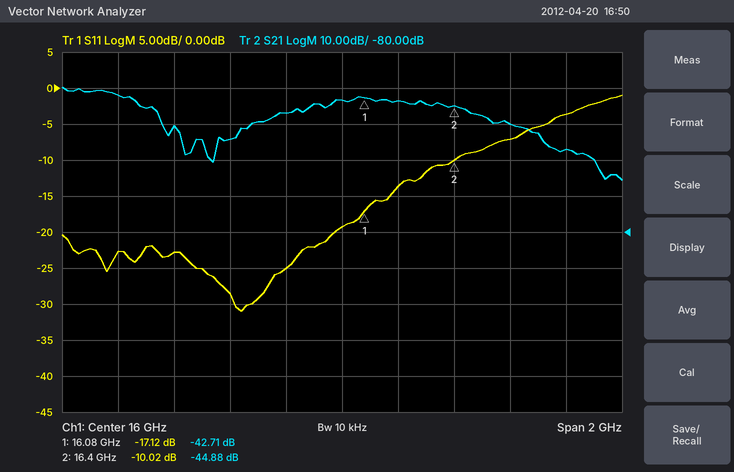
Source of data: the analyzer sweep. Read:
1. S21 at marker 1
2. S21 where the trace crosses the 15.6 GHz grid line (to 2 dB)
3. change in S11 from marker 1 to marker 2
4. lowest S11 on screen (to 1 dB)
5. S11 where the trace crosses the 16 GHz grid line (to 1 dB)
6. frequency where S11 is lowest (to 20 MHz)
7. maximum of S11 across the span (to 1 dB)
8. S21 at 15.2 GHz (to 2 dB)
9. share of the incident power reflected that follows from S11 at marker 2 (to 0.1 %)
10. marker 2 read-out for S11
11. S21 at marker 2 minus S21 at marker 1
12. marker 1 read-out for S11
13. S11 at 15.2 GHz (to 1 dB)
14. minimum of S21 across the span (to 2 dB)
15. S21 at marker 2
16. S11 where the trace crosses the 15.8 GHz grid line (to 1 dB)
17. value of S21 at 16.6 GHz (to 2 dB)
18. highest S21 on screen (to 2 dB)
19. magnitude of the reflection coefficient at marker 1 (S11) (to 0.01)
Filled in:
-42.71 dB
-54 dB
7.10 dB
-31 dB
-19 dB
15.64 GHz
-1 dB
-42 dB
10.0 %
-10.02 dB
-2.17 dB
-17.12 dB
-23 dB
-66 dB
-44.88 dB
-25 dB
-50 dB
-40 dB
0.14
